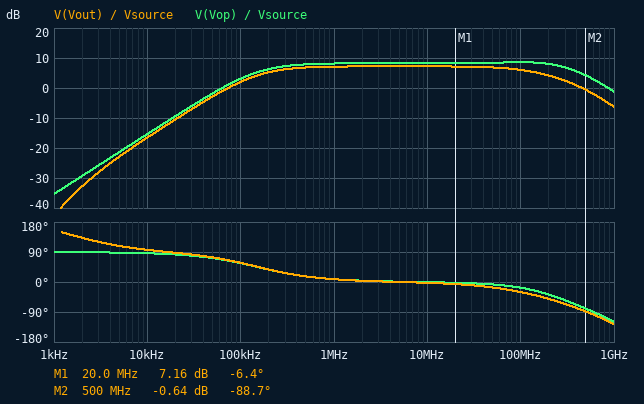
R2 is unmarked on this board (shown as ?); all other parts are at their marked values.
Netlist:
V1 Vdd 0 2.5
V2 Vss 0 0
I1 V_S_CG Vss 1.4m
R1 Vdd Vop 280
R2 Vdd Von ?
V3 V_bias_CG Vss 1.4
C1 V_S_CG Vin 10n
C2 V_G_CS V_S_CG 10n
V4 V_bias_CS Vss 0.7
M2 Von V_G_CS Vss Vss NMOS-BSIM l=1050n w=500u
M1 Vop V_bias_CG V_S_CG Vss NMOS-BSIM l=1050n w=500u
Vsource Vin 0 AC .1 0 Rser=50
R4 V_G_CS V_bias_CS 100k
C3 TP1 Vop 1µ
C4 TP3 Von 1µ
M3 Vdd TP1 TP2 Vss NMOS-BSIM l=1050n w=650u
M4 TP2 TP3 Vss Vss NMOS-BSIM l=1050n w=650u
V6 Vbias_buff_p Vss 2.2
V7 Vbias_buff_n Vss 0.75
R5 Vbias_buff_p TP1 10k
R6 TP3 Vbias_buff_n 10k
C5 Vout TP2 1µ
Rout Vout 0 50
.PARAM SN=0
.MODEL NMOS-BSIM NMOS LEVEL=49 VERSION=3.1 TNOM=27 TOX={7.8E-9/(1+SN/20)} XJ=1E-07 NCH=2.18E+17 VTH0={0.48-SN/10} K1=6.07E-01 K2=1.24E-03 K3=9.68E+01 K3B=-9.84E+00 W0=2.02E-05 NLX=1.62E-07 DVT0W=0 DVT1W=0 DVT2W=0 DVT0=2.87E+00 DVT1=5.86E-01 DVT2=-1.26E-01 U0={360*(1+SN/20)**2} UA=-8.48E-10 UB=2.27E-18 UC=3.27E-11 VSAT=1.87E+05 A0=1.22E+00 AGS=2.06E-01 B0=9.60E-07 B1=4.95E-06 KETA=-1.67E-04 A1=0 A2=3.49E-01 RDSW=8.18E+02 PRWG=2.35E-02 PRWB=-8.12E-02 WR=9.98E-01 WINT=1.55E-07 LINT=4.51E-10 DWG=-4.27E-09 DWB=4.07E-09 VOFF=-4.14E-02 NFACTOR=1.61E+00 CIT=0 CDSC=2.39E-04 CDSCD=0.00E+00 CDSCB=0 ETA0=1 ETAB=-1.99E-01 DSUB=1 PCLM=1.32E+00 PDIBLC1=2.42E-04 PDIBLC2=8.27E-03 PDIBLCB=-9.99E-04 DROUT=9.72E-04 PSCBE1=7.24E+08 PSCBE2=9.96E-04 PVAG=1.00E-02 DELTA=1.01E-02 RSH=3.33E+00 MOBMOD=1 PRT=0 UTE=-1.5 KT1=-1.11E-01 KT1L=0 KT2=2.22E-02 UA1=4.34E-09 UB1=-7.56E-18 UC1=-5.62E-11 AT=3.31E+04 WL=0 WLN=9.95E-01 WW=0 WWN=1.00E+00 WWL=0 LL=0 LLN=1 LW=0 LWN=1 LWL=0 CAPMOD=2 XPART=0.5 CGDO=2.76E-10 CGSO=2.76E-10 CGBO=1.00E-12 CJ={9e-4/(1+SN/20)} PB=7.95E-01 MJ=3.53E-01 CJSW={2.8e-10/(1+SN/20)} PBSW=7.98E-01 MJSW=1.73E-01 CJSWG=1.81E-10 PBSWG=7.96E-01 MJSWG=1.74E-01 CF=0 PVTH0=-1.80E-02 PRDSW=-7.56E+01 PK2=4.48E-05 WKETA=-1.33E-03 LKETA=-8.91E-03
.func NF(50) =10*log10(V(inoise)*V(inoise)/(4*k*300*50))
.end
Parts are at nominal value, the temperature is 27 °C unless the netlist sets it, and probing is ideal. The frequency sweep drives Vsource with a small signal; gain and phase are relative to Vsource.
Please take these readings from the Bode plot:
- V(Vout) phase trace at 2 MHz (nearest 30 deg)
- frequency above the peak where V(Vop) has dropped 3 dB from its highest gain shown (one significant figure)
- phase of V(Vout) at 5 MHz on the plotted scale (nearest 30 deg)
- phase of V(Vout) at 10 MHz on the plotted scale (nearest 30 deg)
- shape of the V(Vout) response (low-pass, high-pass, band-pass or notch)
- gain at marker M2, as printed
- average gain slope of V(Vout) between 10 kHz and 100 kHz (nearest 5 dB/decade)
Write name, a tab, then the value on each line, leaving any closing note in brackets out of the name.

V(Vout) phase trace at 2 MHz	0 deg
frequency above the peak where V(Vop) has dropped 3 dB from its highest gain shown	400 MHz
phase of V(Vout) at 5 MHz on the plotted scale	0 deg
phase of V(Vout) at 10 MHz on the plotted scale	0 deg
shape of the V(Vout) response	band-pass
gain at marker M2, as printed	-0.64 dB
average gain slope of V(Vout) between 10 kHz and 100 kHz	20 dB/decade
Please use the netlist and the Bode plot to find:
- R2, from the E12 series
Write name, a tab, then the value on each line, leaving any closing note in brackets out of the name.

R2, from the E12 series	470 Ω
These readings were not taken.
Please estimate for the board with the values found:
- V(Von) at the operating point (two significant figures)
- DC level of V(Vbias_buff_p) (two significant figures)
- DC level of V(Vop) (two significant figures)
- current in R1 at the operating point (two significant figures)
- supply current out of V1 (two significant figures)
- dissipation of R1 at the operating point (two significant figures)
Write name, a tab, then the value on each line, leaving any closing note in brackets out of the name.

V(Von) at the operating point	2.1 V
DC level of V(Vbias_buff_p)	2.2 V
DC level of V(Vop)	2.1 V
current in R1 at the operating point	1.4 mA
supply current out of V1	4.2 mA
dissipation of R1 at the operating point	550 µW
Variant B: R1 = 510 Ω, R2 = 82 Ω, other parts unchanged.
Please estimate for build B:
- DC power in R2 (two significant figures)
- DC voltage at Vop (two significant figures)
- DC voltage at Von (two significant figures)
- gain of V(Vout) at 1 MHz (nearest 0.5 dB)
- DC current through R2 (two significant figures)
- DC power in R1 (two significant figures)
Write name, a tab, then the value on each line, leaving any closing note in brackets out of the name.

DC power in R2	67 µW
DC voltage at Vop	1.8 V
DC voltage at Von	2.4 V
gain of V(Vout) at 1 MHz	7.0 dB
DC current through R2	910 µA
DC power in R1	1.0 mW
